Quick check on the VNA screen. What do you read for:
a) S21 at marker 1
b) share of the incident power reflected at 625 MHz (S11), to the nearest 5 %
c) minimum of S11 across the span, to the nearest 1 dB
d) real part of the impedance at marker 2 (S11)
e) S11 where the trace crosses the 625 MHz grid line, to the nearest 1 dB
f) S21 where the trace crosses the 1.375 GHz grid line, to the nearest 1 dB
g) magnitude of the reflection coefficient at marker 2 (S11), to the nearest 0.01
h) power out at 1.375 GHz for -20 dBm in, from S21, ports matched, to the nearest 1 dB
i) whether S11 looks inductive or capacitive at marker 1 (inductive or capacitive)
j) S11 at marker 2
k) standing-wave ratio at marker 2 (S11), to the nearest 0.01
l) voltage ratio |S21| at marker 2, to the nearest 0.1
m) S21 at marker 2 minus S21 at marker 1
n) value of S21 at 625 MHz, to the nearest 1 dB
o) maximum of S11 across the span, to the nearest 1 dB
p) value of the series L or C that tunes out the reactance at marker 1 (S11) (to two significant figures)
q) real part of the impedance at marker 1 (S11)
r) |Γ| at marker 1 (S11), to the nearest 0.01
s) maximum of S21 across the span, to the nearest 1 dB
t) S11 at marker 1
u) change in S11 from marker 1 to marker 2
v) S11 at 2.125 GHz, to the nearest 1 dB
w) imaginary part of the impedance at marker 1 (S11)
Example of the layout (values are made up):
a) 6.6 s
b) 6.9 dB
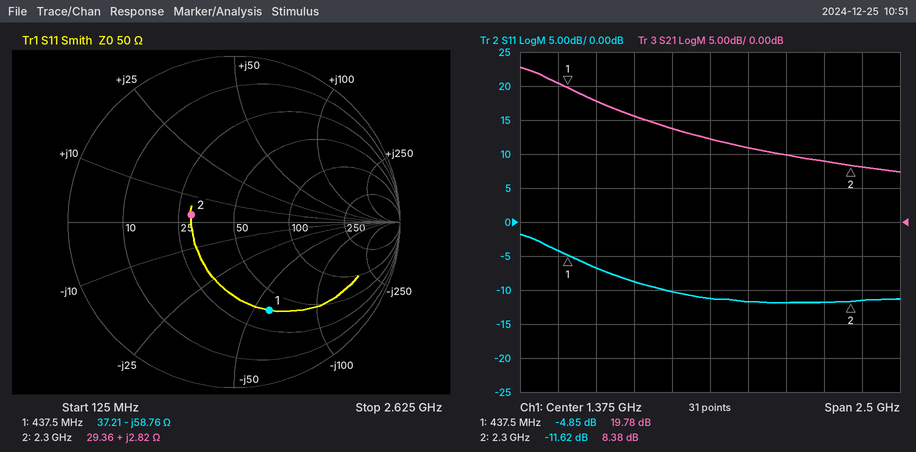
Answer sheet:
a) 19.78 dB
b) 20 %
c) -12 dB
d) 29.36 Ω
e) -7 dB
f) 12 dB
g) 0.26
h) -8 dBm
i) capacitive
j) -11.62 dB
k) 1.71
l) 2.6
m) -11.40 dB
n) 18 dB
o) -2 dB
p) 21 nH
q) 37.21 Ω
r) 0.57
s) 23 dB
t) -4.85 dB
u) -6.77 dB
v) -12 dB
w) -58.76 Ω
